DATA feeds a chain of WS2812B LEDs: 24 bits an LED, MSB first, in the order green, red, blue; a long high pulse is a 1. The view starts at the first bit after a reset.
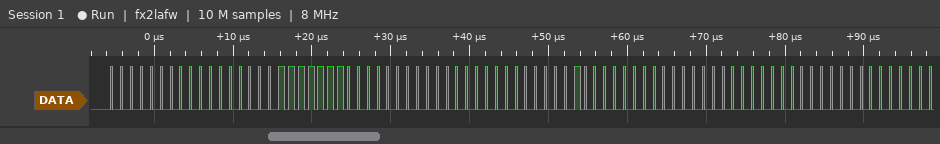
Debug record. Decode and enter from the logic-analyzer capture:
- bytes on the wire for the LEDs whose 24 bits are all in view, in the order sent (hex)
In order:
00 00 7F 00 00 01 00 00 00
